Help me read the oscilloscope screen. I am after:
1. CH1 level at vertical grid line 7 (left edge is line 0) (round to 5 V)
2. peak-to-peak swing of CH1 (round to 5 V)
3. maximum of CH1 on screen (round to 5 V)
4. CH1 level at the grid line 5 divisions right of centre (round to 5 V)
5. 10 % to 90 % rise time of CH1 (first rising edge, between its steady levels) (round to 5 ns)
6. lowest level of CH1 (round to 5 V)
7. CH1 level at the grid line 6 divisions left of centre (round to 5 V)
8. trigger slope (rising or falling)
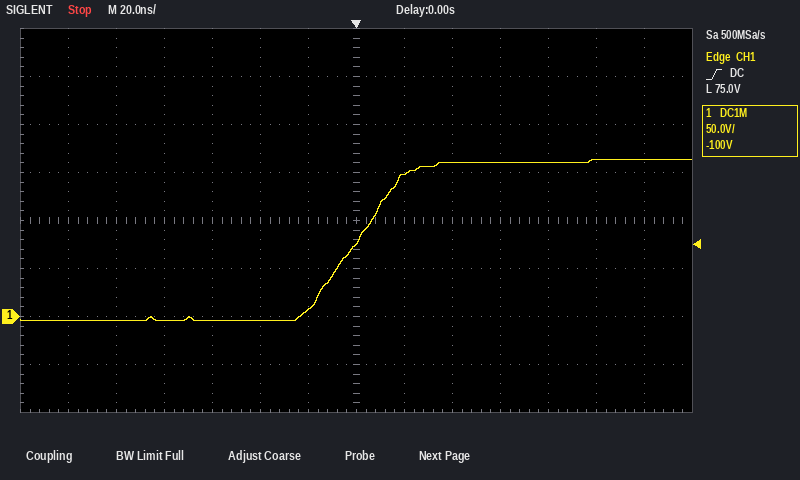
75 V
170 V
165 V
165 V
35 ns
-5 V
-5 V
rising
